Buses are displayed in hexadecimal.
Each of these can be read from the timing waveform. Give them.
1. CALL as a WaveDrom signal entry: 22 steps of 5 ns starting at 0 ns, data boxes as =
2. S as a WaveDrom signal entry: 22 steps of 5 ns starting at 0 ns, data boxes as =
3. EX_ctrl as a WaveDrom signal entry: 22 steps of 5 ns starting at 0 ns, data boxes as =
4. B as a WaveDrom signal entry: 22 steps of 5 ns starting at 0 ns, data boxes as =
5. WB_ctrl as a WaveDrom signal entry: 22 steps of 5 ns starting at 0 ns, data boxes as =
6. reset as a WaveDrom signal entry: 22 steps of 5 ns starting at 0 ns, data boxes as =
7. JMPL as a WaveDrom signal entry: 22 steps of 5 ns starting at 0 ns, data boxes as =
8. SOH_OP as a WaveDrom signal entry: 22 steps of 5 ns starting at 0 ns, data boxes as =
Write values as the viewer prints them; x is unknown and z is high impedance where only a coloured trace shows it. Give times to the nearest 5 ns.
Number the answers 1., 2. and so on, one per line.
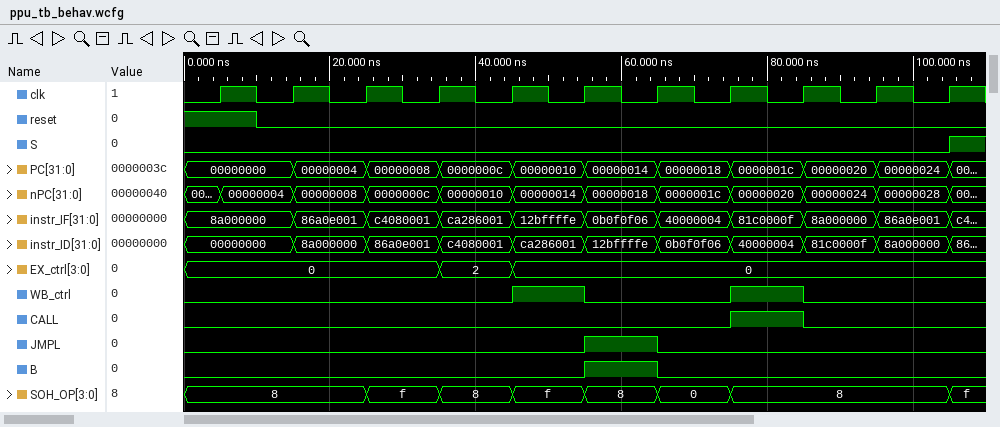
1. {name: 'CALL', wave: '0..............1.0....'}
2. {name: 'S', wave: '0....................1'}
3. {name: 'EX_ctrl', wave: '=......=.=............', data: '0 2 0'}
4. {name: 'B', wave: '0..........1.0........'}
5. {name: 'WB_ctrl', wave: '0........1.0...1.0....'}
6. {name: 'reset', wave: '1.0...................'}
7. {name: 'JMPL', wave: '0..........1.0........'}
8. {name: 'SOH_OP', wave: '=....=.=.=.=.=.=.....=', data: '8 f 8 f 8 0 8 f'}
